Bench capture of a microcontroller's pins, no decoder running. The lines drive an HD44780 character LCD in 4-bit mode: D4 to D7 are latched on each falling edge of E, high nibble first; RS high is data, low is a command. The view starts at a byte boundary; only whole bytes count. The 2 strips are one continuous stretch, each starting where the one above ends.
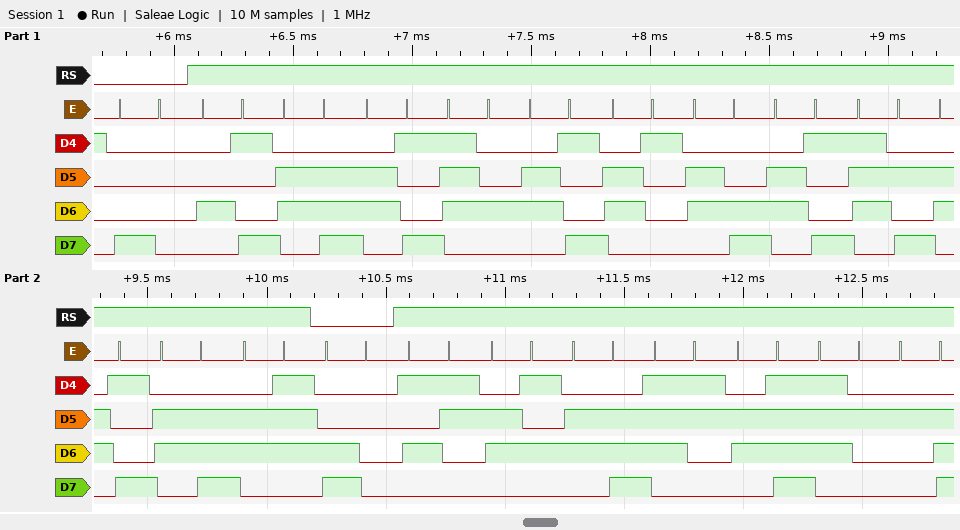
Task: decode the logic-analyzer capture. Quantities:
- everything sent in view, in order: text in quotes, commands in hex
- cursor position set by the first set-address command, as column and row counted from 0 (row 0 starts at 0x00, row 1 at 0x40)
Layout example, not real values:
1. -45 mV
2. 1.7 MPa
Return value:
1. 0x80 "Initializing" 0xC0 "Sensor."
2. column 0, row 0
